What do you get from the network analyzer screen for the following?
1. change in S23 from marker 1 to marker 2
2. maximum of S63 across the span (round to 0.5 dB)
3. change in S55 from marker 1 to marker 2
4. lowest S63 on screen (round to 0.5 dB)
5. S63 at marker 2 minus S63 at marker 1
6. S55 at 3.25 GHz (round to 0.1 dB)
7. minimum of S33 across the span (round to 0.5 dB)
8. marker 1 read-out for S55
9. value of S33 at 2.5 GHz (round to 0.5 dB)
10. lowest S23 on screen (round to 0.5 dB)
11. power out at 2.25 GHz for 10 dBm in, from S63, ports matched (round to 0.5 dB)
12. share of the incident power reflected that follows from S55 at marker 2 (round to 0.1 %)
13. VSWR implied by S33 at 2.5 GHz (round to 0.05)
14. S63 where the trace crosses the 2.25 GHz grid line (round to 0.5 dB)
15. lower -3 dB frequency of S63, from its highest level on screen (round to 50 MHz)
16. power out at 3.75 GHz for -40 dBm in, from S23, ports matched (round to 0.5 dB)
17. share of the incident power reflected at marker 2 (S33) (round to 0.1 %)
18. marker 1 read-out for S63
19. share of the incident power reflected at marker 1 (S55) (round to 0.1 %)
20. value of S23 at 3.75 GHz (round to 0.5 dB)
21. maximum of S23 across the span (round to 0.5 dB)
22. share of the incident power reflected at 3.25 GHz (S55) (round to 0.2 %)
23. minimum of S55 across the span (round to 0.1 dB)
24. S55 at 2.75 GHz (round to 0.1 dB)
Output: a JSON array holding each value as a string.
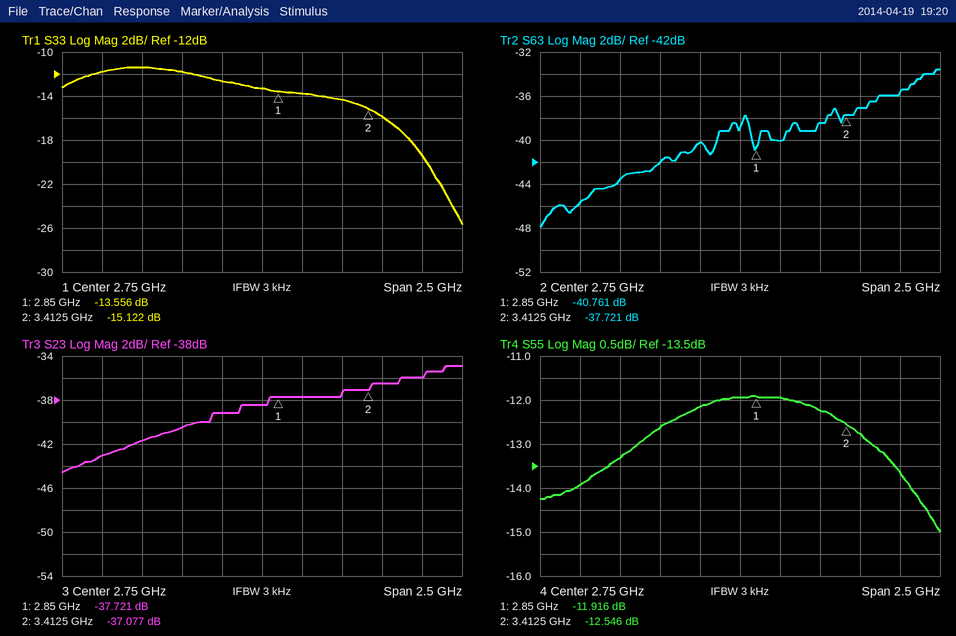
["0.644 dB", "-33.5 dB", "-0.630 dB", "-48.0 dB", "3.040 dB", "-12.2 dB", "-25.5 dB", "-11.916 dB", "-12.5 dB", "-44.5 dB", "-32.0 dBm", "5.6 %", "1.60", "-42.0 dB", "3.55 GHz", "-76.0 dBm", "3.1 %", "-40.761 dB", "6.4 %", "-36.0 dB", "-35.0 dB", "6.0 %", "-15.0 dB", "-11.9 dB"]
